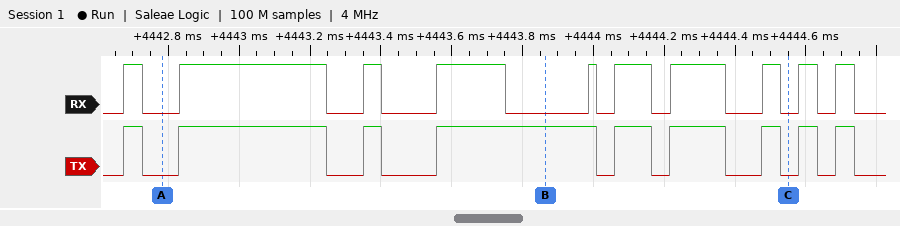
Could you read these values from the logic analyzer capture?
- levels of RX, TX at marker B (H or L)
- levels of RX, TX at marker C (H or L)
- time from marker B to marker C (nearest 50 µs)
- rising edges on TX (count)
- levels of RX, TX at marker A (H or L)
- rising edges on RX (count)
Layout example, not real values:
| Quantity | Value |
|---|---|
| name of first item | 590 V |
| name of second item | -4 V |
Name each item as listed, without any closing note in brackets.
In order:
| Quantity | Value |
|---|---|
| levels of RX, TX at marker B | RX=L, TX=H |
| levels of RX, TX at marker C | RX=L, TX=L |
| time from marker B to marker C | 700 µs |
| rising edges on TX | 9 |
| levels of RX, TX at marker A | RX=L, TX=L |
| rising edges on RX | 10 |
